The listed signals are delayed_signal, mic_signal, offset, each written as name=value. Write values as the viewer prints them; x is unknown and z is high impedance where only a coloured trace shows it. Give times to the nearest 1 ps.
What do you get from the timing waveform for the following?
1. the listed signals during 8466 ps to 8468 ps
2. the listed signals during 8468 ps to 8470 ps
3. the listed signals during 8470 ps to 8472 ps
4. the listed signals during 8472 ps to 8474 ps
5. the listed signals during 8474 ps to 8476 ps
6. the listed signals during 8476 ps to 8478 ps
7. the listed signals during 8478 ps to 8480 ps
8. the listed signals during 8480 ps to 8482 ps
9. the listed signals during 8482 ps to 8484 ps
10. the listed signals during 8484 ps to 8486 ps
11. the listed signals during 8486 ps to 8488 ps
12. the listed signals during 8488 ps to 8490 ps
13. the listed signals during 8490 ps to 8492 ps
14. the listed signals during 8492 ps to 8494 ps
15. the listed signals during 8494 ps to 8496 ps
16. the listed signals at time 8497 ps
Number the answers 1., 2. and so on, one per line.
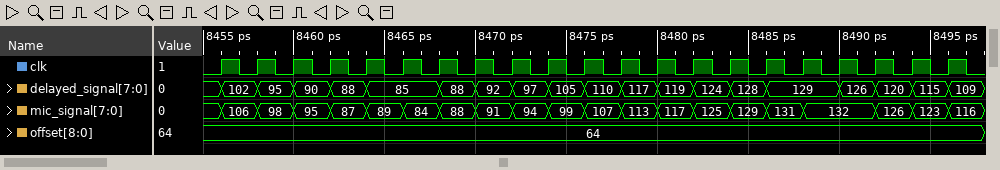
1. delayed_signal=85, mic_signal=84, offset=64
2. delayed_signal=88, mic_signal=88, offset=64
3. delayed_signal=92, mic_signal=91, offset=64
4. delayed_signal=97, mic_signal=94, offset=64
5. delayed_signal=105, mic_signal=99, offset=64
6. delayed_signal=110, mic_signal=107, offset=64
7. delayed_signal=117, mic_signal=113, offset=64
8. delayed_signal=119, mic_signal=117, offset=64
9. delayed_signal=124, mic_signal=125, offset=64
10. delayed_signal=128, mic_signal=129, offset=64
11. delayed_signal=129, mic_signal=131, offset=64
12. delayed_signal=129, mic_signal=132, offset=64
13. delayed_signal=126, mic_signal=132, offset=64
14. delayed_signal=120, mic_signal=126, offset=64
15. delayed_signal=115, mic_signal=123, offset=64
16. delayed_signal=109, mic_signal=116, offset=64
